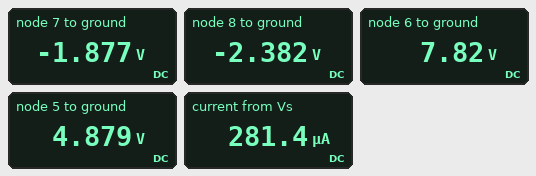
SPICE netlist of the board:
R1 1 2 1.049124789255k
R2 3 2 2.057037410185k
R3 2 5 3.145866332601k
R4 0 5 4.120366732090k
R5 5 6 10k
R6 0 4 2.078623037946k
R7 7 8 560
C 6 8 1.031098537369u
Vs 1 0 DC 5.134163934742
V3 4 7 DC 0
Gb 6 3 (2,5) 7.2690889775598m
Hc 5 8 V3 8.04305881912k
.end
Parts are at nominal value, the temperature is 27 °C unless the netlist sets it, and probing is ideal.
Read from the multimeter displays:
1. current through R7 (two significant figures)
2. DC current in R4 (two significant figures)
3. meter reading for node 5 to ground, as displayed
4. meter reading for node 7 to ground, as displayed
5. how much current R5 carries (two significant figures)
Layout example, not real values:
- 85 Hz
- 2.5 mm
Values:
- 900 µA
- 1.2 mA
- 4.879 V
- -1.877 V
- 290 µA
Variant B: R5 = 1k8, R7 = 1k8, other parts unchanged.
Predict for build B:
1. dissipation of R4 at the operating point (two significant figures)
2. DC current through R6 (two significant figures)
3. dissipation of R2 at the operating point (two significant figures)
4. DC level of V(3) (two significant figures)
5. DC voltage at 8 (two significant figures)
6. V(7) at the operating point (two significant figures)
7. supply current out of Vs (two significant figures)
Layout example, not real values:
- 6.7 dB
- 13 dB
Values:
- 6.4 mW
- 1.2 mA
- 390 nW
- 5.1 V
- -4.8 V
- -2.6 V
- 13 µA
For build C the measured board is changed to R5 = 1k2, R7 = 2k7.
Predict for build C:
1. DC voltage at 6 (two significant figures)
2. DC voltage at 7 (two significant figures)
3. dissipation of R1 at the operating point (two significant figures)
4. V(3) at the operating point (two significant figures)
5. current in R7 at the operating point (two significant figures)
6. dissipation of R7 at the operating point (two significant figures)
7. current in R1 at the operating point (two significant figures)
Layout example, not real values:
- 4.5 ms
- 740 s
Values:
- 5.0 V
- -3.5 V
- 130 µW
- 6.2 V
- 1.7 mA
- 7.5 mW
- 350 µA
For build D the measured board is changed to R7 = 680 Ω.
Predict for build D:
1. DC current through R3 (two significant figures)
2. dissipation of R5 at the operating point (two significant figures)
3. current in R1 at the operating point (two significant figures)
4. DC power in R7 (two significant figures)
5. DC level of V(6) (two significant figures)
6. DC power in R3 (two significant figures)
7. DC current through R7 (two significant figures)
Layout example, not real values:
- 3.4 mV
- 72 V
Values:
- 12 µA
- 750 µW
- 260 µA
- 580 µW
- 7.6 V
- 450 nW
- 930 µA
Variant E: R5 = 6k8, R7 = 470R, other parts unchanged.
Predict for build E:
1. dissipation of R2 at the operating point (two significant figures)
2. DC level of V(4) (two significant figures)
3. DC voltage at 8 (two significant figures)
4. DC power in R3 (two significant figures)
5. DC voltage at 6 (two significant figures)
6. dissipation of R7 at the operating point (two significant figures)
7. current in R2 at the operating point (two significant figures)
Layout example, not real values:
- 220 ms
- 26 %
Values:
- 200 µW
- -1.8 V
- -2.3 V
- 570 nW
- 7.0 V
- 370 µW
- 310 µA
